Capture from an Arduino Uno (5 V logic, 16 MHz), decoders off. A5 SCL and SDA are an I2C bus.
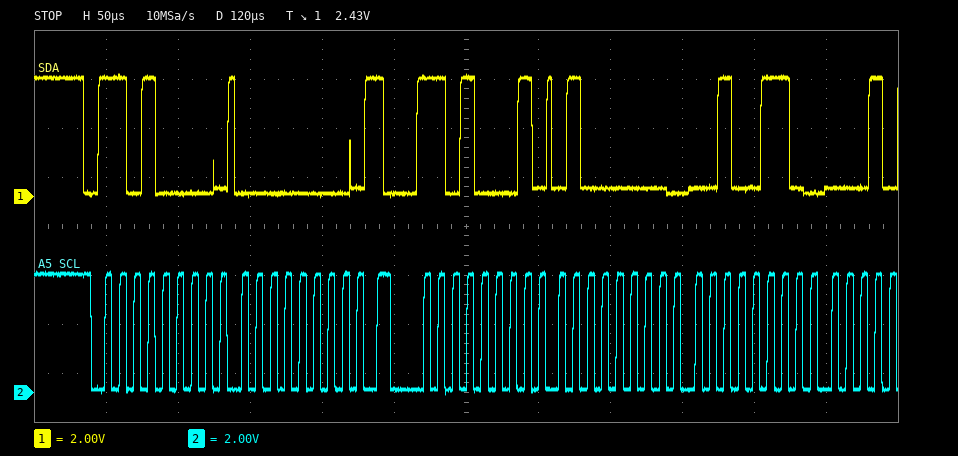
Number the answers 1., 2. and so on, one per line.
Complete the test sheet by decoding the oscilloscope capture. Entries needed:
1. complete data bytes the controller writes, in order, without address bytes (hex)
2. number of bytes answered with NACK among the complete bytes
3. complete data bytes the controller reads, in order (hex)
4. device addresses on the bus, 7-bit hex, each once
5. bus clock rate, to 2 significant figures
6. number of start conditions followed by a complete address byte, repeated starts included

1. 00
2. 0
3. 40 26
4. 0x68
5. 100 kHz
6. 2
